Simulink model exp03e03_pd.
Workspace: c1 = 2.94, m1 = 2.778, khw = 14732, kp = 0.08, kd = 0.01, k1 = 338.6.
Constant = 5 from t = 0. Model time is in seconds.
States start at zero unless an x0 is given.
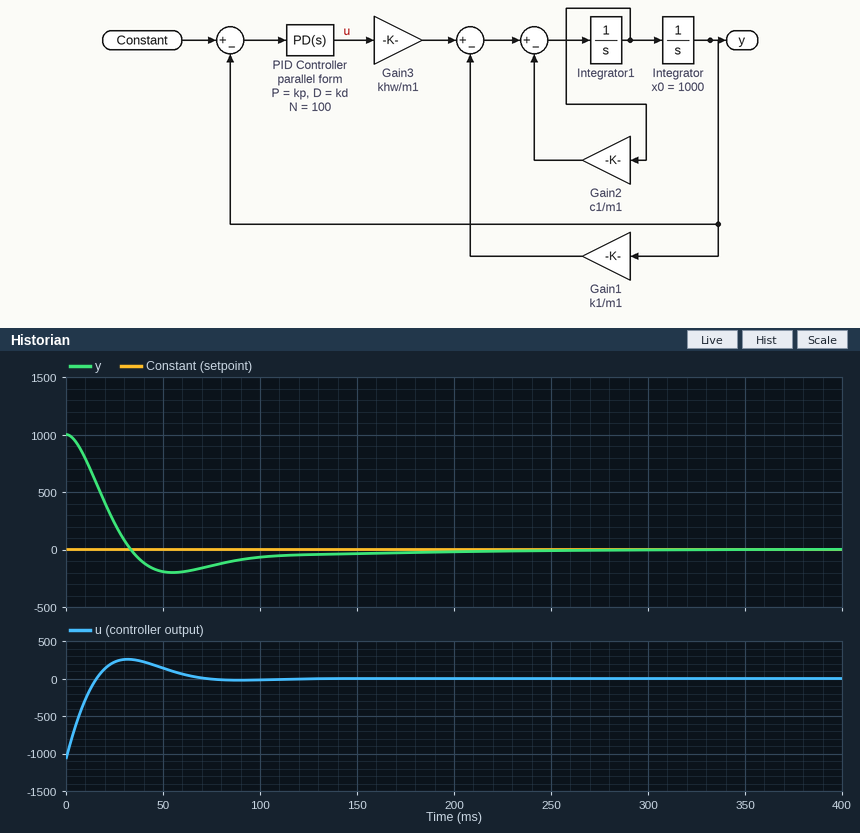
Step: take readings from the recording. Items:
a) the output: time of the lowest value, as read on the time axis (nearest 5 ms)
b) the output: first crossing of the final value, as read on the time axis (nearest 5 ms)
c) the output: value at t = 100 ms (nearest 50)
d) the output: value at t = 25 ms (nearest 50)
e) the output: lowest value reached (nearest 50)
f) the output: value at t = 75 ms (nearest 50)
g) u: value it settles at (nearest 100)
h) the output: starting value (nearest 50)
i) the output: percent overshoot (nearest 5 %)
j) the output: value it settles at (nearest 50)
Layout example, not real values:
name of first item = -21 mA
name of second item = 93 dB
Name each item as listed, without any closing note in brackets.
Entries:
the output: time of the lowest value, as read on the time axis = 55 ms
the output: first crossing of the final value, as read on the time axis = 35 ms
the output: value at t = 100 ms = -50
the output: value at t = 25 ms = 250
the output: lowest value reached = -200
the output: value at t = 75 ms = -150
u: value it settles at = 0
the output: starting value = 1000
the output: percent overshoot = 20 %
the output: value it settles at = 0
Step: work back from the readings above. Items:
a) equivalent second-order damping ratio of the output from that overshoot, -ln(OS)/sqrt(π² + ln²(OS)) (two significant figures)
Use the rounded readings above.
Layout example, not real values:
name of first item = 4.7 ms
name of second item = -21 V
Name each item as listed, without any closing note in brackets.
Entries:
equivalent second-order damping ratio of the output from that overshoot, -ln(OS)/sqrt(π² + ln²(OS)) = 0.46
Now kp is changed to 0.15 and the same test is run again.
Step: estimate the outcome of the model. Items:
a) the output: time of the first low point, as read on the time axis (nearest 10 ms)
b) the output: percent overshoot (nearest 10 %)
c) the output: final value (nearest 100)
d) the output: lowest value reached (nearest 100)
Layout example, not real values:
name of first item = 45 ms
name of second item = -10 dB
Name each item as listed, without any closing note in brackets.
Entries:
the output: time of the first low point, as read on the time axis = 50 ms
the output: percent overshoot = 30 %
the output: final value = 0
the output: lowest value reached = -300
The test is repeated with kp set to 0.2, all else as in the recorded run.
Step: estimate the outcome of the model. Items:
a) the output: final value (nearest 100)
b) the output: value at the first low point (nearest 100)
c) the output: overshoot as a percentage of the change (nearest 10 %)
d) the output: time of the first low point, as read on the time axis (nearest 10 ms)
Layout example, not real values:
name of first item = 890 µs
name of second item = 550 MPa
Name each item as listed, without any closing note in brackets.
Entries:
the output: final value = 0
the output: value at the first low point = -300
the output: overshoot as a percentage of the change = 30 %
the output: time of the first low point, as read on the time axis = 50 ms
